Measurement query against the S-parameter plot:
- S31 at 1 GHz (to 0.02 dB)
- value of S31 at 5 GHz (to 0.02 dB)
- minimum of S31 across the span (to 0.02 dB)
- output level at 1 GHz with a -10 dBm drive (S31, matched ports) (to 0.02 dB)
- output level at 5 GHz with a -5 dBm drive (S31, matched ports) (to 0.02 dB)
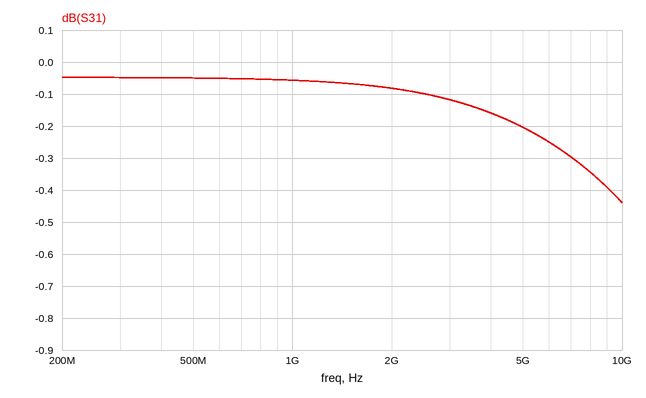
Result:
-0.06 dB
-0.20 dB
-0.44 dB
-10.06 dBm
-5.20 dBm
